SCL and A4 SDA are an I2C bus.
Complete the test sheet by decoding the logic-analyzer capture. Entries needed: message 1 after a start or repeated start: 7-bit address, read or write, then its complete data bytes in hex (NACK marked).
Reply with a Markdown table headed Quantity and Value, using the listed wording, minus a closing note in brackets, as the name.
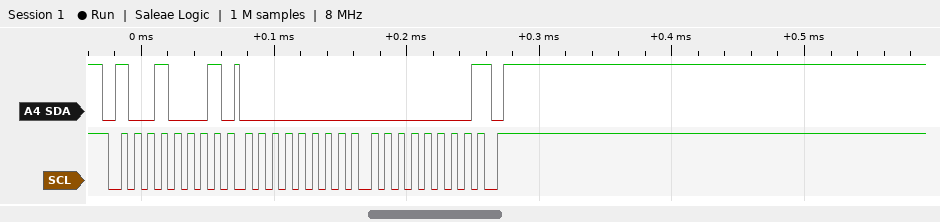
| Quantity | Value |
|---|---|
| message 1 after a start or repeated start: 7-bit address, read or write, then its complete data bytes in hex | 0x48 read: 00 00 NACK |
